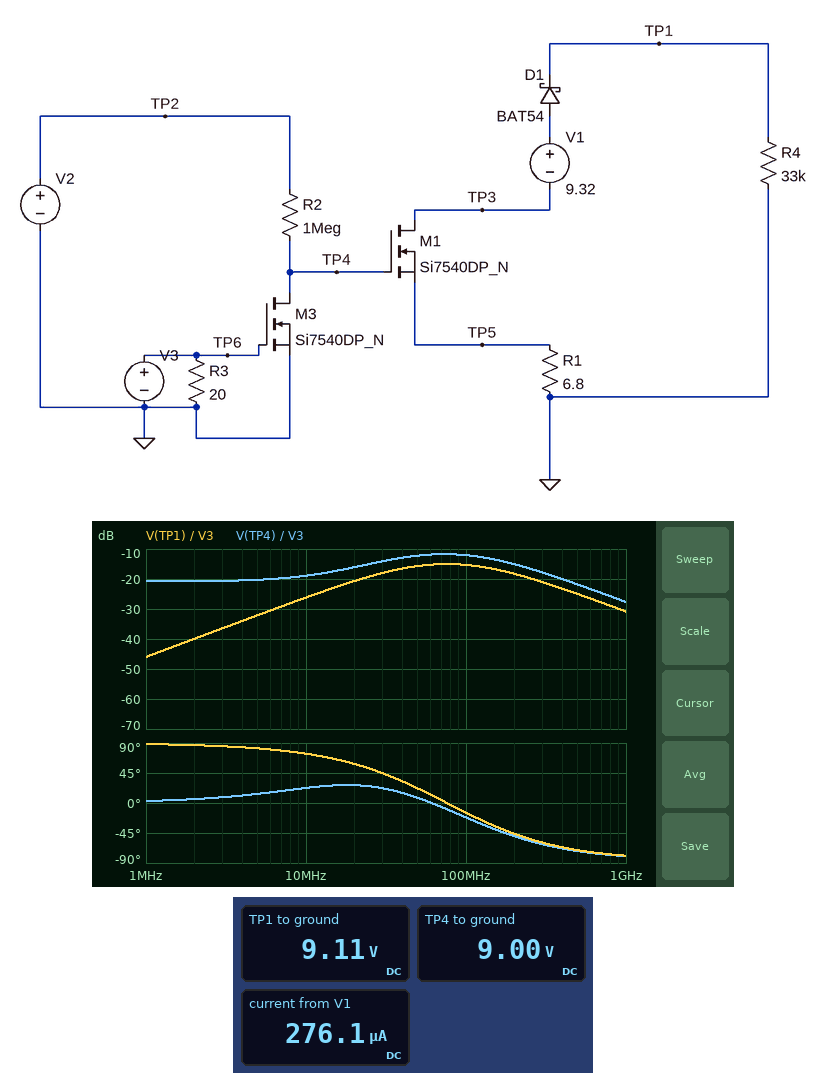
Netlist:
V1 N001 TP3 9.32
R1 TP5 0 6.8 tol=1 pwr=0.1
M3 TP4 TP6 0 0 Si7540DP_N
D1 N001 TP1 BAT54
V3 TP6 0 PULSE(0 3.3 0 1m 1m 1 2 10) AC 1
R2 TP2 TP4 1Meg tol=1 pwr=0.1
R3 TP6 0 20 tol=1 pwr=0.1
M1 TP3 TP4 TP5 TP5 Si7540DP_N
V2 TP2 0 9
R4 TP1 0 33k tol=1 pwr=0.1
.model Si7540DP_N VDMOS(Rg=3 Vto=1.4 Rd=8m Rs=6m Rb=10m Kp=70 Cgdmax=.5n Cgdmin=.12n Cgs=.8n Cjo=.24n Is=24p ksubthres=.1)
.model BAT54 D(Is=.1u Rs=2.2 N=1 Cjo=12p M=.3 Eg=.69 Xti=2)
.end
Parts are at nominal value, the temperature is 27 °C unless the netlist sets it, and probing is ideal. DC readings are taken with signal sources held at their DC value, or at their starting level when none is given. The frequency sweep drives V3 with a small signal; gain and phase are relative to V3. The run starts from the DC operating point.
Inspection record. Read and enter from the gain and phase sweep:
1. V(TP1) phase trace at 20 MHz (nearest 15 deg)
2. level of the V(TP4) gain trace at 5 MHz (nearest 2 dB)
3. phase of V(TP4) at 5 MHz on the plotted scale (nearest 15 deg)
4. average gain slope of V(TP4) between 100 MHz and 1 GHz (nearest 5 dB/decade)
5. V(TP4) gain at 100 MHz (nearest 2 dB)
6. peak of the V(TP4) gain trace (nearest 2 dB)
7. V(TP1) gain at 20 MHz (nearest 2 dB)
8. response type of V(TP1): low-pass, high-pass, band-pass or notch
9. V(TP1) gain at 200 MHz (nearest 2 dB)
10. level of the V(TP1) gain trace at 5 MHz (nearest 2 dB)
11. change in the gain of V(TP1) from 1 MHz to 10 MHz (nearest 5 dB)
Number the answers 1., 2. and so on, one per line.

1. 60 deg
2. -20 dB
3. 15 deg
4. -15 dB/decade
5. -12 dB
6. -12 dB
7. -20 dB
8. band-pass
9. -18 dB
10. -32 dB
11. 20 dB
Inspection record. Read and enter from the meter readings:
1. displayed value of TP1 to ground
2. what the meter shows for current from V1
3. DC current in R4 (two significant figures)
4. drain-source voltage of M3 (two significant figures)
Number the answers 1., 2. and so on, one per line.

1. 9.11 V
2. 276.1 µA
3. 280 µA
4. 9.0 V
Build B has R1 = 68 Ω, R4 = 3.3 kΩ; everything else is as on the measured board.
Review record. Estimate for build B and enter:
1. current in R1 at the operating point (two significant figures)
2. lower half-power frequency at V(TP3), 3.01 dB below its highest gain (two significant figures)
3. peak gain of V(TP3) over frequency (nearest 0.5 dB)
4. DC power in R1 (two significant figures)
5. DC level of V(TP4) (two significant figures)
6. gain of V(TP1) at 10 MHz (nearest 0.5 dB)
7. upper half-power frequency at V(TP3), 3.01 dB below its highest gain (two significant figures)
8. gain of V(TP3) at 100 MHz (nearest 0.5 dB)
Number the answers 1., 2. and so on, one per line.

1. 2.7 mA
2. 9.4 MHz
3. -5.5 dB
4. 490 µW
5. 9.0 V
6. -8.5 dB
7. 86 MHz
8. -9.5 dB
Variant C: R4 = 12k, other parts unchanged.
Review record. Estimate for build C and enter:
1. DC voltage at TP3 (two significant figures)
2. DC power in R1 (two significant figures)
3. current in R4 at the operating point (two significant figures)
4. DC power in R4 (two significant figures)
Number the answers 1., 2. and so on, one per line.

1. -5.2 mV
2. 3.9 µW
3. 760 µA
4. 6.9 mW
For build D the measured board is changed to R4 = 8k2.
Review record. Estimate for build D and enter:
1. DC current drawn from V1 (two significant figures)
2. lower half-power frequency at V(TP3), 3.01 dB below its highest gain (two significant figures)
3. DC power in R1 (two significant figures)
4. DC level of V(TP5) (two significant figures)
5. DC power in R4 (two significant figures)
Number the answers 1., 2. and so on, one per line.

1. 1.1 mA
2. 30 MHz
3. 8.3 µW
4. -7.5 mV
5. 10 mW
